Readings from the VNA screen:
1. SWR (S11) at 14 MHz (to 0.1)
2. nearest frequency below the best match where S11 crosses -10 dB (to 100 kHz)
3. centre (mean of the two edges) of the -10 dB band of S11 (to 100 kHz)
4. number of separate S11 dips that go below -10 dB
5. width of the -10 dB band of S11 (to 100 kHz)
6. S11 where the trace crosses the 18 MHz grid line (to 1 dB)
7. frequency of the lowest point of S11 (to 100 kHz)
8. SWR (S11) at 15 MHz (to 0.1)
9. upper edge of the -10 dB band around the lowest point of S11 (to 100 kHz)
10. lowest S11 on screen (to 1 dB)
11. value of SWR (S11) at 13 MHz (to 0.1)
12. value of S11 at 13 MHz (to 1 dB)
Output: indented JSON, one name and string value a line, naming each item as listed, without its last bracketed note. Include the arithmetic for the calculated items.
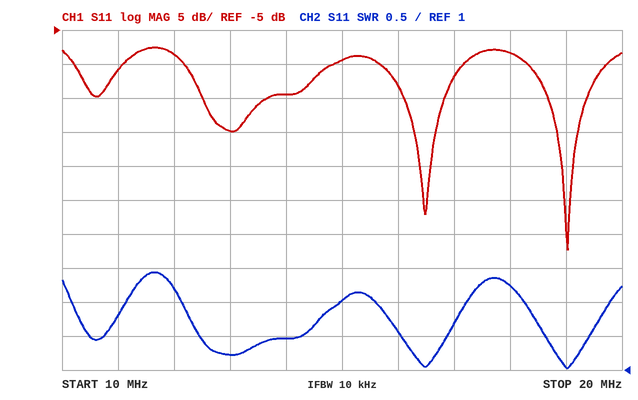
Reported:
{
  "SWR (S11) at 14 MHz": "1.5",
  "nearest frequency below the best match where S11 crosses -10 dB": "18.3 MHz",
  "centre (mean of the two edges) of the -10 dB band of S11": "19.0 MHz",
  "number of separate S11 dips that go below -10 dB": "4",
  "width of the -10 dB band of S11": "19.7 MHz − 18.3 MHz = 1.4 MHz",
  "S11 where the trace crosses the 18 MHz grid line": "-8 dB",
  "frequency of the lowest point of S11": "19.0 MHz",
  "SWR (S11) at 15 MHz": "2.0",
  "upper edge of the -10 dB band around the lowest point of S11": "19.7 MHz",
  "lowest S11 on screen": "-37 dB",
  "value of SWR (S11) at 13 MHz": "1.2",
  "value of S11 at 13 MHz": "-20 dB"
}
